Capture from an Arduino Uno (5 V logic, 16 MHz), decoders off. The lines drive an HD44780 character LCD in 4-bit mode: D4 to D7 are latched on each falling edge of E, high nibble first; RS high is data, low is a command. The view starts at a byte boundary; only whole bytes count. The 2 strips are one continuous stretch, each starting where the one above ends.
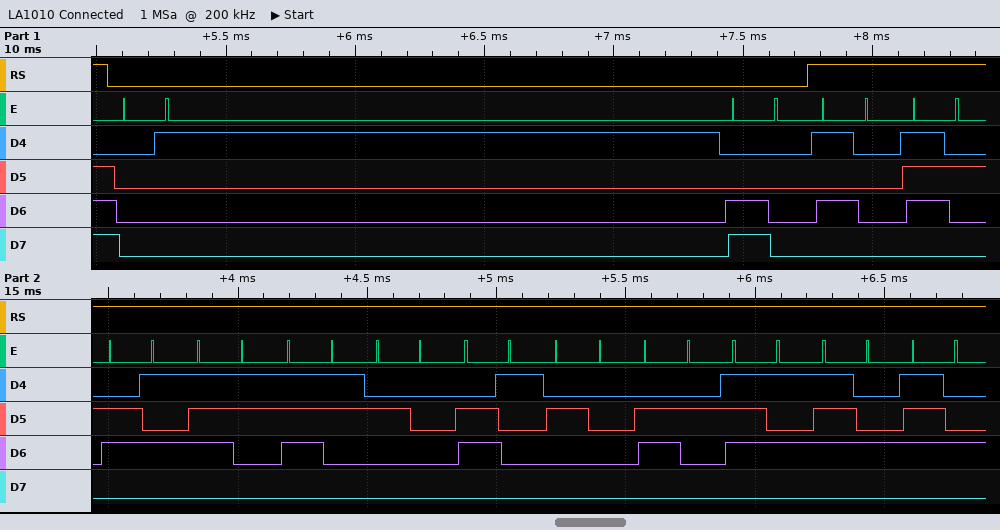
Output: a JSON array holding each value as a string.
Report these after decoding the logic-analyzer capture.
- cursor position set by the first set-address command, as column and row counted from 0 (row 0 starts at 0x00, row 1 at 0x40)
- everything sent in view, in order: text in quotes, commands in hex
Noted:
["column 0, row 1", "0x01 0xC0 \"Press a butt\""]
